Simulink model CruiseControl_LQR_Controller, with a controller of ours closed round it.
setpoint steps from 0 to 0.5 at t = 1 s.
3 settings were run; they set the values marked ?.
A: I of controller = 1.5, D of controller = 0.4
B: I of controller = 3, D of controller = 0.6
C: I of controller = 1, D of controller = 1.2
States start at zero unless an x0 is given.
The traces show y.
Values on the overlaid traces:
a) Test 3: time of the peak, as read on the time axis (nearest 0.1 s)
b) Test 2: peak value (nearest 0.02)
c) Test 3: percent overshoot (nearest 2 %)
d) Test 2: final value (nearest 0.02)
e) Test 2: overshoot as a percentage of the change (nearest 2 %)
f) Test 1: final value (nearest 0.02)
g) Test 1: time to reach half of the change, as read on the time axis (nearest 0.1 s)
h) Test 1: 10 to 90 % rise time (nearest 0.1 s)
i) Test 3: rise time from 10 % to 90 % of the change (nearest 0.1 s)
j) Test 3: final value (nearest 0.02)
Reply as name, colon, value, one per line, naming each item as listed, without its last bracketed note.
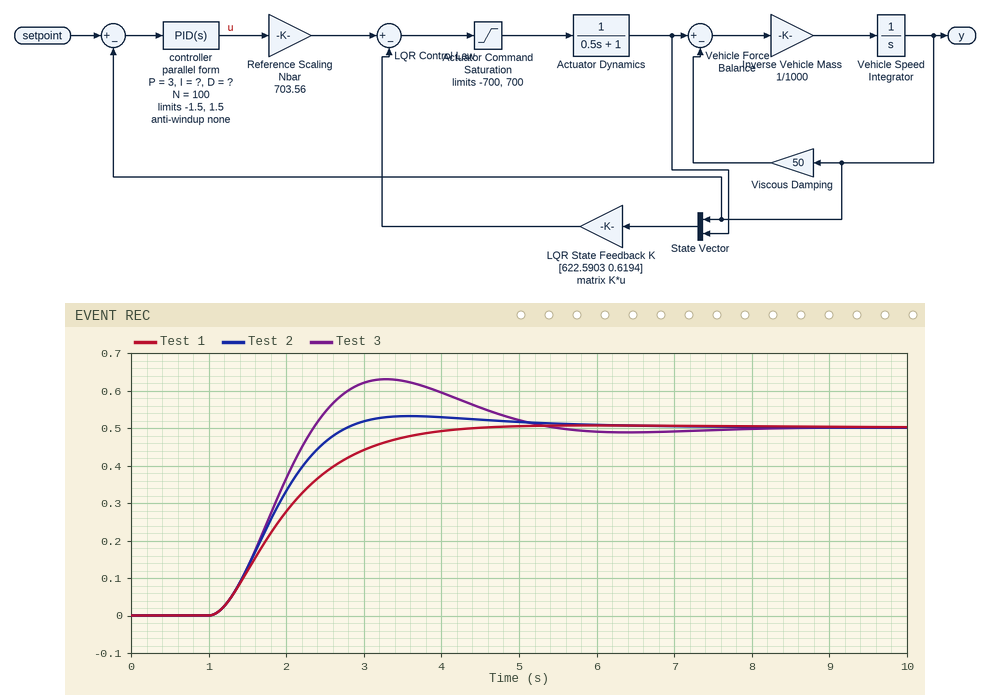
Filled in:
Test 3: time of the peak, as read on the time axis: 3.3 s
Test 2: peak value: 0.54
Test 3: percent overshoot: 26 %
Test 2: final value: 0.50
Test 2: overshoot as a percentage of the change: 6 %
Test 1: final value: 0.50
Test 1: time to reach half of the change, as read on the time axis: 1.9 s
Test 1: 10 to 90 % rise time: 1.8 s
Test 3: rise time from 10 % to 90 % of the change: 0.9 s
Test 3: final value: 0.50
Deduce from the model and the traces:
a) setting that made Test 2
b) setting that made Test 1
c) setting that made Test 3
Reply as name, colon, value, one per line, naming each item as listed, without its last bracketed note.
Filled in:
setting that made Test 2: A
setting that made Test 1: C
setting that made Test 3: B
